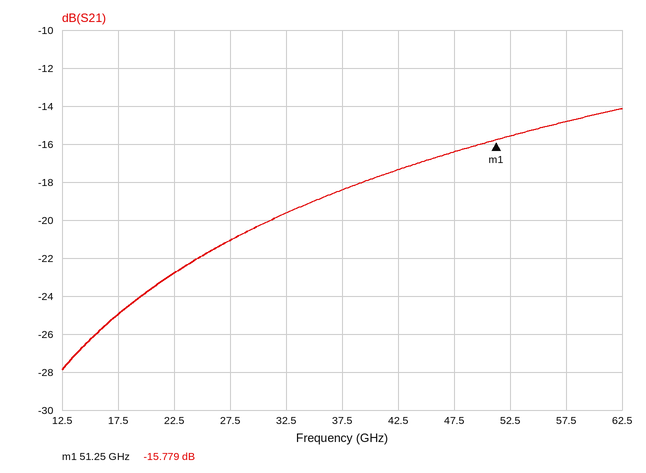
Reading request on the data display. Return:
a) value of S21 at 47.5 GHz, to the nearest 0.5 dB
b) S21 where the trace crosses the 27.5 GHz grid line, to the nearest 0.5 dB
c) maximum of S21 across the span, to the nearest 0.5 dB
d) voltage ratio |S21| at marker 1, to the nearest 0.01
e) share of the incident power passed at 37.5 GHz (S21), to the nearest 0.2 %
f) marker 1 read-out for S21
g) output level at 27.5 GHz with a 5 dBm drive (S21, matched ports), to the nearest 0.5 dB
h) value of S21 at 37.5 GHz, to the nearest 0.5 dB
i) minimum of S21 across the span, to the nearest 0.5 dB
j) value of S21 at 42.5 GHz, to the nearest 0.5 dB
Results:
-16.5 dB
-21.0 dB
-14.0 dB
0.16
1.4 %
-15.779 dB
-16.0 dBm
-18.5 dB
-28.0 dB
-17.5 dB
